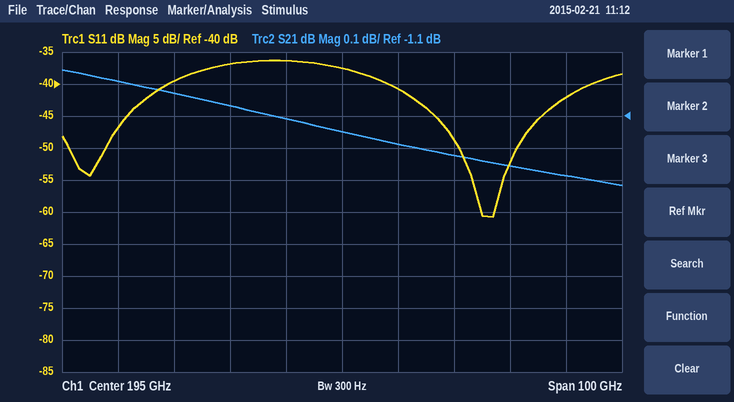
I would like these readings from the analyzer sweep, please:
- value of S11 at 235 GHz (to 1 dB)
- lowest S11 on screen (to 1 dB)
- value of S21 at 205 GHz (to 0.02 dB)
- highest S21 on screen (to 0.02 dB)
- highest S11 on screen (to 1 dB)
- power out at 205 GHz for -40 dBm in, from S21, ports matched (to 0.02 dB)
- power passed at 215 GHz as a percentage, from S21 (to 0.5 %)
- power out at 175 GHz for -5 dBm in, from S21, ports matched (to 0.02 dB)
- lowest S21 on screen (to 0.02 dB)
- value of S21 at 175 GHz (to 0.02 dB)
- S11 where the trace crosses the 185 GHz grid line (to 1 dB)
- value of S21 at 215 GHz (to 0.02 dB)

-42 dB
-61 dB
-1.18 dB
-0.96 dB
-36 dB
-41.18 dBm
75.5 %
-6.06 dBm
-1.32 dB
-1.06 dB
-36 dB
-1.22 dB
